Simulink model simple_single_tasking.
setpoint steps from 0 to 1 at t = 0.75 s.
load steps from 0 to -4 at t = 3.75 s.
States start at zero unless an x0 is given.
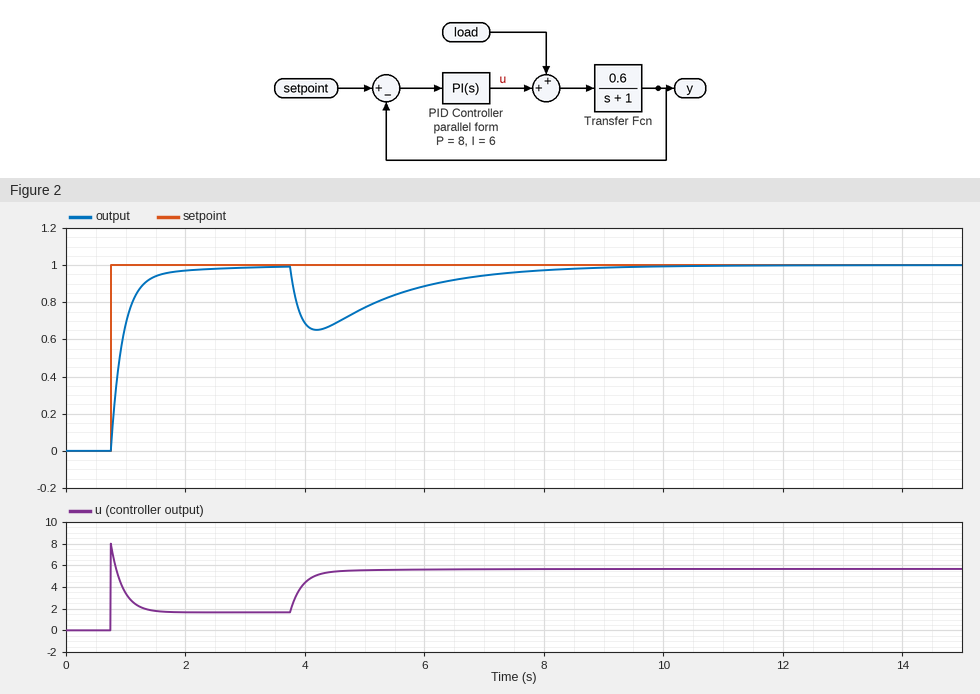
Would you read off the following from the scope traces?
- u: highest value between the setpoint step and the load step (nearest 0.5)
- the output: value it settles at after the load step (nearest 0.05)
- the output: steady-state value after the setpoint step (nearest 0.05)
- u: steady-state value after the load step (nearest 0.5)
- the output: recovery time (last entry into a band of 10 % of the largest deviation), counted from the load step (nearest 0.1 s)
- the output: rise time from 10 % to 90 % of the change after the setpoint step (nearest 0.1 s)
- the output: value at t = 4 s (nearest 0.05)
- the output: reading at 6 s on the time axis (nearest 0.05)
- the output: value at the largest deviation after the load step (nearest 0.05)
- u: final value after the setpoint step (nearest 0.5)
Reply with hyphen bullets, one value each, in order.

- 8.0
- 1.00
- 1.00
- 5.5
- 4.0 s
- 0.5 s
- 0.70
- 0.90
- 0.65
- 1.5
